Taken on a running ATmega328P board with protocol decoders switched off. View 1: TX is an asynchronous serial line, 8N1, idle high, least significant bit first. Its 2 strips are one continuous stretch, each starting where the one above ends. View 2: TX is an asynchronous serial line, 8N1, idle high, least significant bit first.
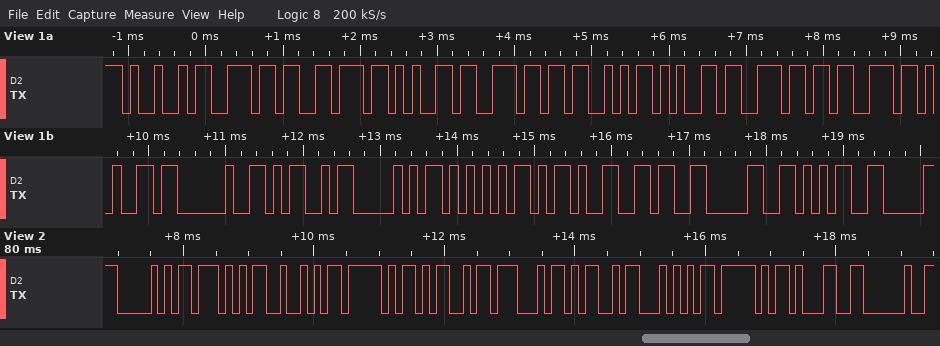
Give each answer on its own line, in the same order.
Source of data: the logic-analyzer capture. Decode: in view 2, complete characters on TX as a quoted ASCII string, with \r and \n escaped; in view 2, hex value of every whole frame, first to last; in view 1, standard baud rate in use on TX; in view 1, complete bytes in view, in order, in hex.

"PWR_MGMT_1 "
50 57 52 5F 4D 47 4D 54 5F 31 20
9600 baud
49 6E 76 65 6E 53 65 6E 73 65 20 4D 50 55 2D 36 30 35
